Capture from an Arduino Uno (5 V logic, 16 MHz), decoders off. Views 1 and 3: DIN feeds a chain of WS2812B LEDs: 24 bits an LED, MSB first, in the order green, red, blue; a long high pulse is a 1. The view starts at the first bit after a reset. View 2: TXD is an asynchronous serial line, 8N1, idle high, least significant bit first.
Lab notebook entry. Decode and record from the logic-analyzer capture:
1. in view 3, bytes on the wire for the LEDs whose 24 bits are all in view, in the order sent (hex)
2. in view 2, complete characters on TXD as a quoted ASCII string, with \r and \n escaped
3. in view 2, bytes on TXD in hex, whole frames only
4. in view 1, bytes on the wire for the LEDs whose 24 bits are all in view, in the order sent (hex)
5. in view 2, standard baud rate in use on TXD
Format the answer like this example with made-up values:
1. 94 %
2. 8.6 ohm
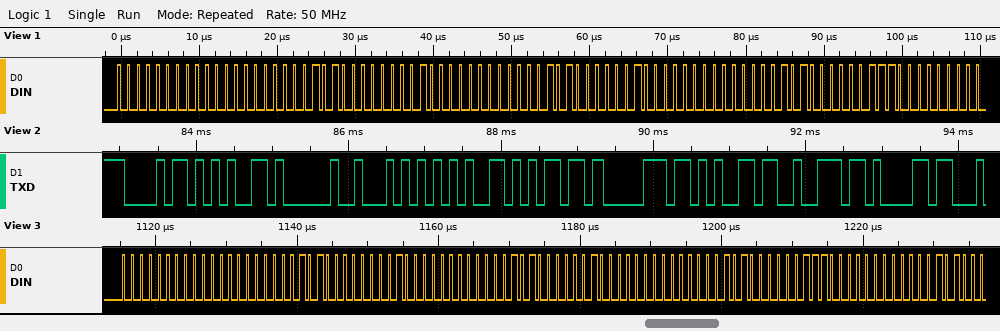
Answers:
1. 00 00 0A 01 00 0A 04 00 0A 07 00 0A
2. "he Tempera"
3. 68 65 20 54 65 6D 70 65 72 61
4. 00 00 0A 01 00 0A 04 00 0A
5. 9600 baud
